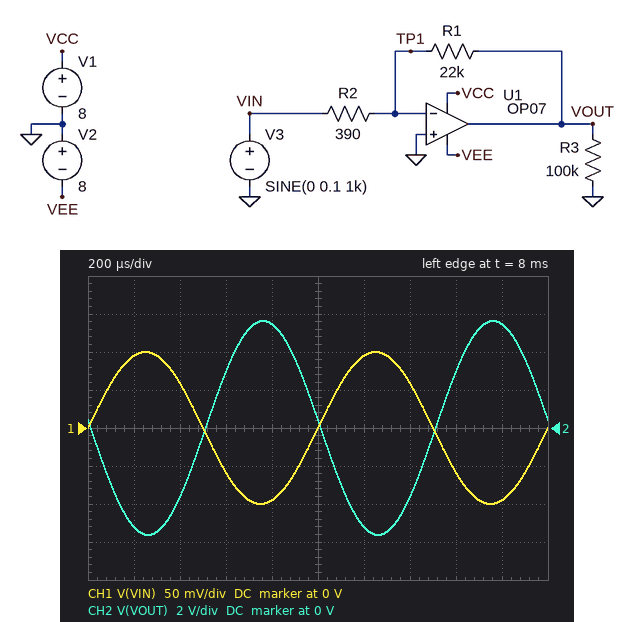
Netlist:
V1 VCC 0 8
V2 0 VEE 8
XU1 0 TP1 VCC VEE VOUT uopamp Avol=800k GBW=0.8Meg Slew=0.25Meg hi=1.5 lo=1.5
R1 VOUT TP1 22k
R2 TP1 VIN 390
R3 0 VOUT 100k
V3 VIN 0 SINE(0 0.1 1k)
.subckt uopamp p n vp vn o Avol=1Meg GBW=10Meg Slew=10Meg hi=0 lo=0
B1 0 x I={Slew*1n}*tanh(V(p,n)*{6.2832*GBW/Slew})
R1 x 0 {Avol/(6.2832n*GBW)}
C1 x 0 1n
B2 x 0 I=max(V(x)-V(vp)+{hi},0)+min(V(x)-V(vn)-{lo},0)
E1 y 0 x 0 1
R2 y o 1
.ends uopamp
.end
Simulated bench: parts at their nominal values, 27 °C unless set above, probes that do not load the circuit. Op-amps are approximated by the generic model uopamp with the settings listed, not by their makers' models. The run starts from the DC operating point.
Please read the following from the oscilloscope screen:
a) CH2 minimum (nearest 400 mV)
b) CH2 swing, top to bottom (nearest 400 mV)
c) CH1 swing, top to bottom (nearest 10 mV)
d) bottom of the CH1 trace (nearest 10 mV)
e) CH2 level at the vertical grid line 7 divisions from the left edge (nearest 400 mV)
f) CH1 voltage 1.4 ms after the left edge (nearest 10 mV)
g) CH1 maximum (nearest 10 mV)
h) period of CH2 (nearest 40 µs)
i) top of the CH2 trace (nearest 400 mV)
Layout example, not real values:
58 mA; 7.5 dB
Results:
-5.6 V; 11.2 V; 200 mV; -100 mV; -3.6 V; 60 mV; 100 mV; 1.00 ms; 5.6 V
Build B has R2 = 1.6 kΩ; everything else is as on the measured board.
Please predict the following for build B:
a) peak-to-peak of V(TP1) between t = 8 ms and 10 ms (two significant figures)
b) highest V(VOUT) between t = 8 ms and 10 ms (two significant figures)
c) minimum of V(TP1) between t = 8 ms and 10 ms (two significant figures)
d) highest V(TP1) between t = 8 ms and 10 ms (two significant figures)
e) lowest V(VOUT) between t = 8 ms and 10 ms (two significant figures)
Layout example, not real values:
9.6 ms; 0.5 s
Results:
3.4 mV; 1.4 V; -1.7 mV; 1.7 mV; -1.4 V
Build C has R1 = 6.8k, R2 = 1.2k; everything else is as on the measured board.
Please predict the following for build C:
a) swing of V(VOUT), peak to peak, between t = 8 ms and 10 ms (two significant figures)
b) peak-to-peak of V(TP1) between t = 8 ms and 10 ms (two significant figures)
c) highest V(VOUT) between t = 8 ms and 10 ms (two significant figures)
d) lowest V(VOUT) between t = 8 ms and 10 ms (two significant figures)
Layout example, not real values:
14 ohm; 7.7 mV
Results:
1.1 V; 1.4 mV; 570 mV; -570 mV
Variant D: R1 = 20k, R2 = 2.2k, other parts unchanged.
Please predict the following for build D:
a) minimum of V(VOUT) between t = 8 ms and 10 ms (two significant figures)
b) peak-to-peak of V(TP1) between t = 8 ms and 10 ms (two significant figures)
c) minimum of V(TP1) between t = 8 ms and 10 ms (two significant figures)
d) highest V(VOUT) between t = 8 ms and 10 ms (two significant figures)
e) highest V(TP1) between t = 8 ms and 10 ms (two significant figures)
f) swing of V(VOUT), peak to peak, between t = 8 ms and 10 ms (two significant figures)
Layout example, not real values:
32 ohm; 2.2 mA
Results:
-910 mV; 2.3 mV; -1.1 mV; 910 mV; 1.1 mV; 1.8 V
